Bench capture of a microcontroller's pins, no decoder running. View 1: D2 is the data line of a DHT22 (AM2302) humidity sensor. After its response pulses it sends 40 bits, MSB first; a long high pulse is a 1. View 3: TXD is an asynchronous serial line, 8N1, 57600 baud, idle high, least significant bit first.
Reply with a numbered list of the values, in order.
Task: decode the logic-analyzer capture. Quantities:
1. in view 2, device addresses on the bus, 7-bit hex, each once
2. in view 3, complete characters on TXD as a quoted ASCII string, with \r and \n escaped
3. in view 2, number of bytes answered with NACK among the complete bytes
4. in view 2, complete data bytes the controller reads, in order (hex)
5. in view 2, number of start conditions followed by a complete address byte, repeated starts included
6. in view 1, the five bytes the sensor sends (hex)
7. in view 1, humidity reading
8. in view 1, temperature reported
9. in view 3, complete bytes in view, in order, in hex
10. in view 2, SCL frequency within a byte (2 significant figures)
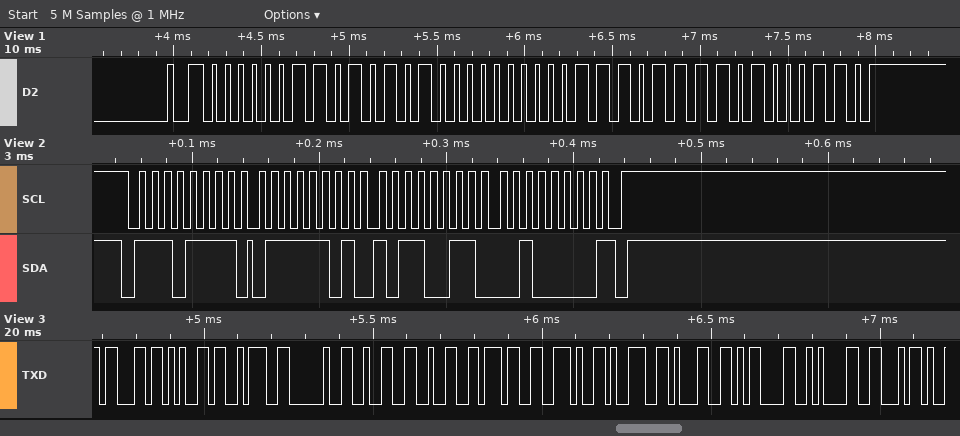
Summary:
1. 0x77
2. "ce: 227.91\r\nF"
3. 1
4. 7D B3 20
5. 1
6. 03 54 00 EF 46
7. 85.2 %
8. 23.9 °C
9. 63 65 3A 20 32 32 37 2E 39 31 0D 0A 46
10. 100 kHz
